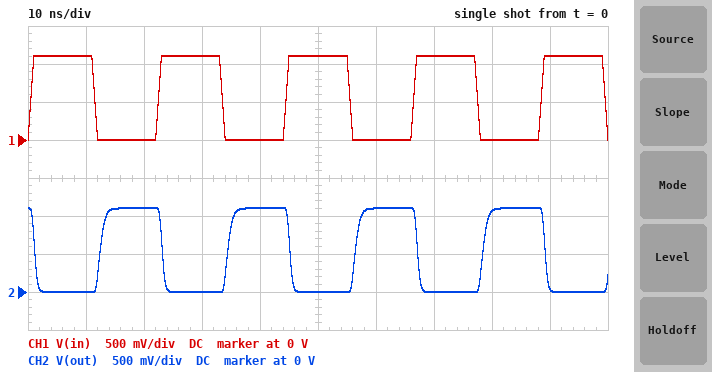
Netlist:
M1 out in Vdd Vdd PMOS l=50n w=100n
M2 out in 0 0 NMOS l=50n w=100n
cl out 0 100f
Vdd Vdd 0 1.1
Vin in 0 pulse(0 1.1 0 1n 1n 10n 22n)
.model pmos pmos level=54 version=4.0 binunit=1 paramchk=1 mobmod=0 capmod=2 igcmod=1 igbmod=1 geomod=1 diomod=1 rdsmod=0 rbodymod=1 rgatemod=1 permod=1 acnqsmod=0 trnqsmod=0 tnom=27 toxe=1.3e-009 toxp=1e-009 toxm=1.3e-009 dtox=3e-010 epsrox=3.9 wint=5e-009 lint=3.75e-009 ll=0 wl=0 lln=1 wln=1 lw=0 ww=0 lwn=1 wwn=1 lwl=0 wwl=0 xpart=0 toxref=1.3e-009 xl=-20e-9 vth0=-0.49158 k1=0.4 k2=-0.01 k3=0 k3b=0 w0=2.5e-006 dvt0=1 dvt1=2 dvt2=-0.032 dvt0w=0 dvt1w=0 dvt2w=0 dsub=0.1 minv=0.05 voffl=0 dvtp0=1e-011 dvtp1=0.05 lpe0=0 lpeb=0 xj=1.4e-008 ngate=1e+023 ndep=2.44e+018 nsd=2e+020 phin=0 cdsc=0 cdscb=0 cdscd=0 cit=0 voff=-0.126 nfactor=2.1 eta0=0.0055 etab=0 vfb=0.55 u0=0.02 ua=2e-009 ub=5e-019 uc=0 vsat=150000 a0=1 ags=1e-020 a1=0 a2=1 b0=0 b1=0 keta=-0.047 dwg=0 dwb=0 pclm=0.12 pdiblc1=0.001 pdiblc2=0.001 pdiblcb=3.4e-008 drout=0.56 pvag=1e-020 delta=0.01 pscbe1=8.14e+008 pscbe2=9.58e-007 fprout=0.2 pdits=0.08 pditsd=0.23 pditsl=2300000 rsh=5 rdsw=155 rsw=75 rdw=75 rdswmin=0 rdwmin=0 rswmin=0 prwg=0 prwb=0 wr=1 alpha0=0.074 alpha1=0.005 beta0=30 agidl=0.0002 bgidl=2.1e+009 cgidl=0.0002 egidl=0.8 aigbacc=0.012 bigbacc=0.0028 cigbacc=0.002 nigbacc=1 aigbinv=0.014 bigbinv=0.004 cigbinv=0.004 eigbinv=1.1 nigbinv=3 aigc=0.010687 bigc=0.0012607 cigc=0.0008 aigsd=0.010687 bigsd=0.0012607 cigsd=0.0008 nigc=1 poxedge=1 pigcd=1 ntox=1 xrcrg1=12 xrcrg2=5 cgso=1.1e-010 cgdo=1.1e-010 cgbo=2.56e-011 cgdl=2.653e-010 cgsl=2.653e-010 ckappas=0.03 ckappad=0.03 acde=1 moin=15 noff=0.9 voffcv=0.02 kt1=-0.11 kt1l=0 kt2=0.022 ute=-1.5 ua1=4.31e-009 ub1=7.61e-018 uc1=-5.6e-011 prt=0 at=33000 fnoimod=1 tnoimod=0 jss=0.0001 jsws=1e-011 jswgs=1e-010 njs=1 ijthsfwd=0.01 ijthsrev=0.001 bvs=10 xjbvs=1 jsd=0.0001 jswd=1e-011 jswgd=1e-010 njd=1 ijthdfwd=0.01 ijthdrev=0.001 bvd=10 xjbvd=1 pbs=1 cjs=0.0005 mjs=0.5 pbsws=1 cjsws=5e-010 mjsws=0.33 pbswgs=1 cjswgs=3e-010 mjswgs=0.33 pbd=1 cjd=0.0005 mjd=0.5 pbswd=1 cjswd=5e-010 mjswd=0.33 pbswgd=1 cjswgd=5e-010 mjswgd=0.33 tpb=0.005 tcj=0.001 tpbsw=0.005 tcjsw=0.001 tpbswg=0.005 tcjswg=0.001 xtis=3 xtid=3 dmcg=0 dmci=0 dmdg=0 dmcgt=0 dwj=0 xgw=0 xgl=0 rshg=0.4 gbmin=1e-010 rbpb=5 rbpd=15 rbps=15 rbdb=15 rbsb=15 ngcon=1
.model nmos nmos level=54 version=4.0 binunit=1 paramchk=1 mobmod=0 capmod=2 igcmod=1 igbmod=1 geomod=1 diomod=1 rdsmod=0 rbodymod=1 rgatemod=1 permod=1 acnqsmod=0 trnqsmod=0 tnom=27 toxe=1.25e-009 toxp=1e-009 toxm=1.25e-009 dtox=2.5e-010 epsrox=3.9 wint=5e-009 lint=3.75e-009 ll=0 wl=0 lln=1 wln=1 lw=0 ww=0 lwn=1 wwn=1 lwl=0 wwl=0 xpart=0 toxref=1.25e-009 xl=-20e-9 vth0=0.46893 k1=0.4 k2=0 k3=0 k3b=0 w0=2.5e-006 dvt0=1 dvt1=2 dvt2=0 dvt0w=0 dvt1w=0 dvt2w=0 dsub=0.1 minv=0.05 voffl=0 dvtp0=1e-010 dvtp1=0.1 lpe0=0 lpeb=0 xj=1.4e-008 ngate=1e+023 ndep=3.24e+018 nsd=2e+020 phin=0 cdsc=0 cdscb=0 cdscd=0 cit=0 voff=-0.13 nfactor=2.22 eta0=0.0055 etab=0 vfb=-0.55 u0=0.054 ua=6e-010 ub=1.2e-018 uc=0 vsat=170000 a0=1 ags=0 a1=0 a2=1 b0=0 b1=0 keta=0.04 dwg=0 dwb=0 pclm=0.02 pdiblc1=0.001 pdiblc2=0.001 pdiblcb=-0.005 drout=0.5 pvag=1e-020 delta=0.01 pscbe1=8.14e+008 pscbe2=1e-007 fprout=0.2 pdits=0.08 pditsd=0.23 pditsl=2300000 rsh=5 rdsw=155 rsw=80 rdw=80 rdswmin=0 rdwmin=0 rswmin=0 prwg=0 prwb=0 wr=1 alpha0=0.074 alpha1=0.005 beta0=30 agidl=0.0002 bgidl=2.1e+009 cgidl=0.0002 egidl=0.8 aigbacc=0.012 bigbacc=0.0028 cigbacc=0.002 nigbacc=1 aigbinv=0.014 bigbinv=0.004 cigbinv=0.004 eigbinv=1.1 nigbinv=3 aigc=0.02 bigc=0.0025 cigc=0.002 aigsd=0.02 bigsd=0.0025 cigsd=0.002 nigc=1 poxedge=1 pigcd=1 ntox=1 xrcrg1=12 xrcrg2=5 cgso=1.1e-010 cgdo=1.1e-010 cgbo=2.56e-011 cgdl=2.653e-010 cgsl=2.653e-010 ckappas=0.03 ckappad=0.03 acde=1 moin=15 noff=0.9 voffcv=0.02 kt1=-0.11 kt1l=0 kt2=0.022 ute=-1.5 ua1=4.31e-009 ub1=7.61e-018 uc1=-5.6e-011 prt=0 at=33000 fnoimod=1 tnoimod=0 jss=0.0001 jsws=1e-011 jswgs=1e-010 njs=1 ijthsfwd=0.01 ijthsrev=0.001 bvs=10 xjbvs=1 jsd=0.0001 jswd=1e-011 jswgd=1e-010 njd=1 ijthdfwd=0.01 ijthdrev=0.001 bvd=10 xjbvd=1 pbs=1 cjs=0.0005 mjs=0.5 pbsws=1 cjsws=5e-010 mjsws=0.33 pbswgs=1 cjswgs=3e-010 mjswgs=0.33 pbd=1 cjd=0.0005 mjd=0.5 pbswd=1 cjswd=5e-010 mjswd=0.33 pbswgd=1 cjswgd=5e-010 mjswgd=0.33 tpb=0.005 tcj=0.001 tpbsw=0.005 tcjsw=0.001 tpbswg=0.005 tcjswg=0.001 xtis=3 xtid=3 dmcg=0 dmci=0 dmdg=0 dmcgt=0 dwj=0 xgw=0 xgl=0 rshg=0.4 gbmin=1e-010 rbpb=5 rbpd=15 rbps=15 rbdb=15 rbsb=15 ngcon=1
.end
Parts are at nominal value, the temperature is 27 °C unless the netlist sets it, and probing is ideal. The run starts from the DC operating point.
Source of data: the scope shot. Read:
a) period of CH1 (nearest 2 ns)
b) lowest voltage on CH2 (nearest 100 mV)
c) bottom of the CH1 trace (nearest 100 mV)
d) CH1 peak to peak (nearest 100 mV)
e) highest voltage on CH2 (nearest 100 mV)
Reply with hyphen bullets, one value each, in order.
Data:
- 22 ns
- 0 V
- 0 V
- 1.1 V
- 1.1 V
